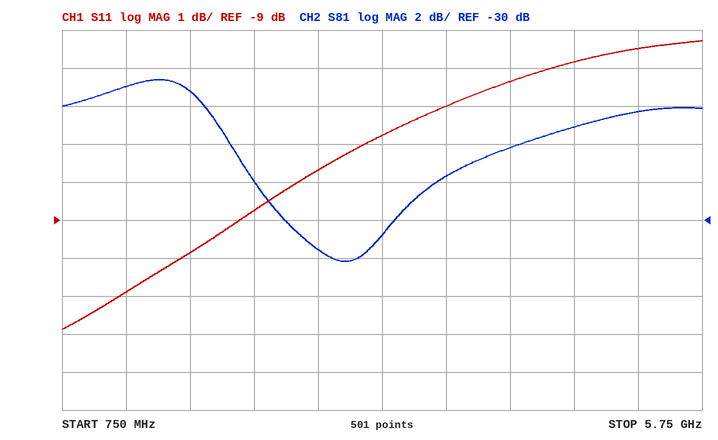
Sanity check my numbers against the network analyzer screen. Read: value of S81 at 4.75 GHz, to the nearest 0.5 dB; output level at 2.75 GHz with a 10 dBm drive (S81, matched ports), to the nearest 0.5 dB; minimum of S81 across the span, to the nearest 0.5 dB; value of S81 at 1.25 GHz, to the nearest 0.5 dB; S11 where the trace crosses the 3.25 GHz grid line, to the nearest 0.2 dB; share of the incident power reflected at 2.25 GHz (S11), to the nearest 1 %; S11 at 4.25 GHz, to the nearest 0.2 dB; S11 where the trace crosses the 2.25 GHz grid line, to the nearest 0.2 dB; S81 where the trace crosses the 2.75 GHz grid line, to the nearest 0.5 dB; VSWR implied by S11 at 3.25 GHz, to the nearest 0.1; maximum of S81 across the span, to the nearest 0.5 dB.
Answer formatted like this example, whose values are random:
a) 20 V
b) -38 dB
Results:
a) -25.0 dB
b) -21.5 dBm
c) -32.0 dB
d) -23.0 dB
e) -6.8 dB
f) 13 %
g) -5.4 dB
h) -8.8 dB
i) -31.5 dB
j) 2.7
k) -22.5 dB
